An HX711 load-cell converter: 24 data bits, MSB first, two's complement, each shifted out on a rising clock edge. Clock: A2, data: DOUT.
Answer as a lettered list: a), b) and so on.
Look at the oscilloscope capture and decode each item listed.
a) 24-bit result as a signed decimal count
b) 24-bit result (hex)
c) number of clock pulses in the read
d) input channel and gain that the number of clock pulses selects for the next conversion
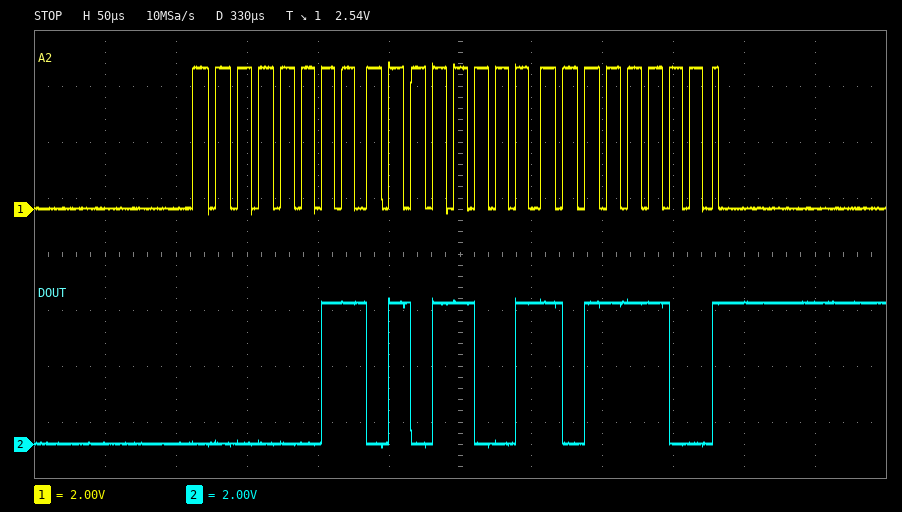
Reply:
a) 219580
b) 0x0359BC
c) 25
d) channel A, gain 128
